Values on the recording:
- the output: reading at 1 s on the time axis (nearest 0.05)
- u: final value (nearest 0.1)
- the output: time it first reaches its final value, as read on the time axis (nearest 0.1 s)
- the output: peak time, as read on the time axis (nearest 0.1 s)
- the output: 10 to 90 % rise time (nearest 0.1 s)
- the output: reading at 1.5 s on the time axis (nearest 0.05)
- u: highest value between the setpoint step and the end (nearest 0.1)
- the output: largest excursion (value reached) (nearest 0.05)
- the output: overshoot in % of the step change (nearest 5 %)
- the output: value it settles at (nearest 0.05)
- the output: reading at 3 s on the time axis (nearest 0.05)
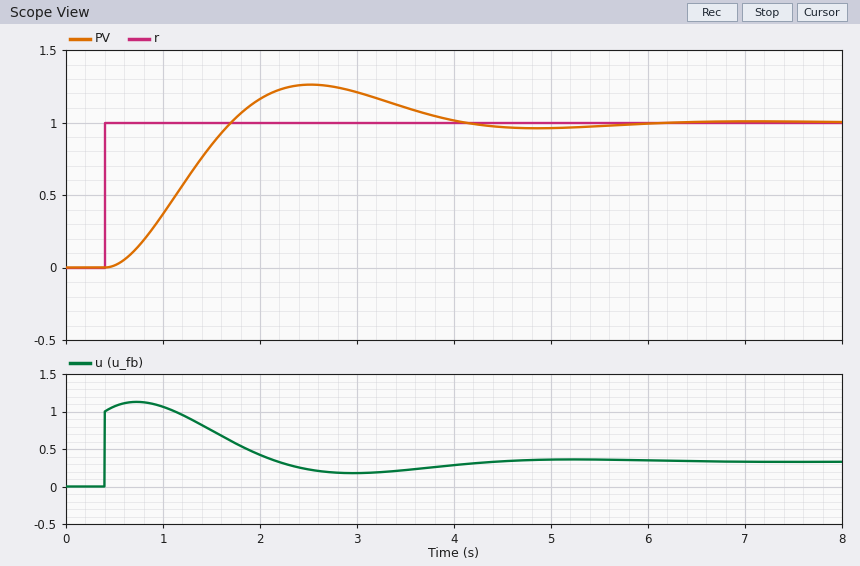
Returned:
0.35
0.3
1.7 s
2.5 s
0.9 s
0.85
1.1
1.25
25 %
1.00
1.20
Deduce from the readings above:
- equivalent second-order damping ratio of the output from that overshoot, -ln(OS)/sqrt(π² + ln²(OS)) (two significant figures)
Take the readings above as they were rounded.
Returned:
0.40
